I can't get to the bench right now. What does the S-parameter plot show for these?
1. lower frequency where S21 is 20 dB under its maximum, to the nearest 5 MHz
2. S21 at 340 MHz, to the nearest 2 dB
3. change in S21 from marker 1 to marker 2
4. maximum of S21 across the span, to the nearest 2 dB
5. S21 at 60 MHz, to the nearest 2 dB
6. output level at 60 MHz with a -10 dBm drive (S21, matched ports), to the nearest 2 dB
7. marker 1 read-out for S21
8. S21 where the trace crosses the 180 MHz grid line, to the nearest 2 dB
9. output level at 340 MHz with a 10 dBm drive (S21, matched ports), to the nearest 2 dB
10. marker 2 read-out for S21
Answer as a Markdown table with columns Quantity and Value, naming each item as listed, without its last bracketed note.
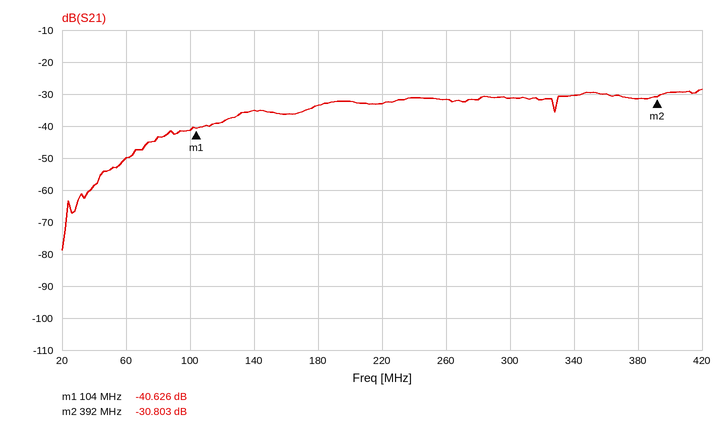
| Quantity | Value |
|---|---|
| lower frequency where S21 is 20 dB under its maximum, to the nearest 5 MHz | 65 MHz |
| S21 at 340 MHz, to the nearest 2 dB | -30 dB |
| change in S21 from marker 1 to marker 2 | 9.823 dB |
| maximum of S21 across the span, to the nearest 2 dB | -28 dB |
| S21 at 60 MHz, to the nearest 2 dB | -50 dB |
| output level at 60 MHz with a -10 dBm drive (S21, matched ports), to the nearest 2 dB | -60 dBm |
| marker 1 read-out for S21 | -40.626 dB |
| S21 where the trace crosses the 180 MHz grid line, to the nearest 2 dB | -34 dB |
| output level at 340 MHz with a 10 dBm drive (S21, matched ports), to the nearest 2 dB | -20 dBm |
| marker 2 read-out for S21 | -30.803 dB |
